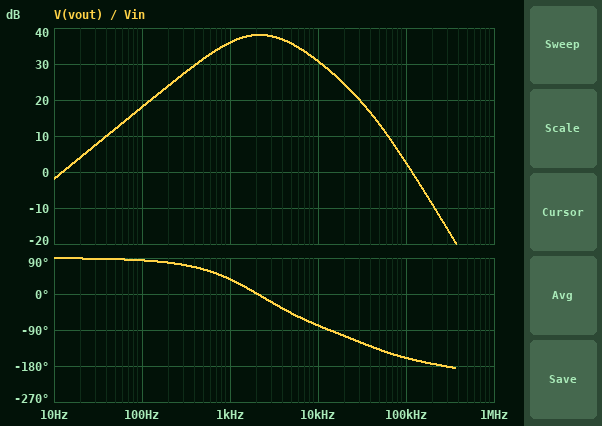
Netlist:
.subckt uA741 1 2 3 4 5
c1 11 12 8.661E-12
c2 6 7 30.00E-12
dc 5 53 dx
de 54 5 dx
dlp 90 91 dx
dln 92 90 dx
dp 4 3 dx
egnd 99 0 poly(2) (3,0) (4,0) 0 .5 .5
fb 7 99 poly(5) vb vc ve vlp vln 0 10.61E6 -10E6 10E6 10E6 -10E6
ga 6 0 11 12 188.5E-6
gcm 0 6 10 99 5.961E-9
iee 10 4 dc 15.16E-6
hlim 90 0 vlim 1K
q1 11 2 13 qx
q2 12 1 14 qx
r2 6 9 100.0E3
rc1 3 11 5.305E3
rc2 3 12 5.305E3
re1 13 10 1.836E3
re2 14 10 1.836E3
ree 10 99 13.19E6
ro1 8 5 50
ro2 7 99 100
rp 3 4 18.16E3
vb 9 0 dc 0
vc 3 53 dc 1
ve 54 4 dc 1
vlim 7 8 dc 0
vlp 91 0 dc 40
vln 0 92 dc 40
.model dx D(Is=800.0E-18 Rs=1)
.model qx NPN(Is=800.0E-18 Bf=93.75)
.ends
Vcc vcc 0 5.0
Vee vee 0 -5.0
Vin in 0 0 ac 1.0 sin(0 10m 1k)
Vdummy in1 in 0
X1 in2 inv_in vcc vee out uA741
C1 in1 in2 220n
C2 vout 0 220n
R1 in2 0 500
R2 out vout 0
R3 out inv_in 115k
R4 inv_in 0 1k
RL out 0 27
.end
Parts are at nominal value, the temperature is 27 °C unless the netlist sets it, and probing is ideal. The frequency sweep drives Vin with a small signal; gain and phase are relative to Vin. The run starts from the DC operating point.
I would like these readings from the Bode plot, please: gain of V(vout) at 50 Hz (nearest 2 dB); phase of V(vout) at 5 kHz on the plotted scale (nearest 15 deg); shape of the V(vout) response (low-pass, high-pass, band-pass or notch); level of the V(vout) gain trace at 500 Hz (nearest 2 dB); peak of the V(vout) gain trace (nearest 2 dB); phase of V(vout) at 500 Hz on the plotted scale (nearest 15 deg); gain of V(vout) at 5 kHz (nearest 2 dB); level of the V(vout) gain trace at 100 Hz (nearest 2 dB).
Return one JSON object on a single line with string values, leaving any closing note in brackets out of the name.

{"gain of V(vout) at 50 Hz": "12 dB", "phase of V(vout) at 5 kHz on the plotted scale": "-45 deg", "shape of the V(vout) response": "band-pass", "level of the V(vout) gain trace at 500 Hz": "32 dB", "peak of the V(vout) gain trace": "38 dB", "phase of V(vout) at 500 Hz on the plotted scale": "60 deg", "gain of V(vout) at 5 kHz": "36 dB", "level of the V(vout) gain trace at 100 Hz": "18 dB"}
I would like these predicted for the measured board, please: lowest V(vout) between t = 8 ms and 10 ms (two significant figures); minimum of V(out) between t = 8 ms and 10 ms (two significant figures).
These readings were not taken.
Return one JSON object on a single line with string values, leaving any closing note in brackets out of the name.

{"lowest V(vout) between t = 8 ms and 10 ms": "-620 mV", "minimum of V(out) between t = 8 ms and 10 ms": "-620 mV"}
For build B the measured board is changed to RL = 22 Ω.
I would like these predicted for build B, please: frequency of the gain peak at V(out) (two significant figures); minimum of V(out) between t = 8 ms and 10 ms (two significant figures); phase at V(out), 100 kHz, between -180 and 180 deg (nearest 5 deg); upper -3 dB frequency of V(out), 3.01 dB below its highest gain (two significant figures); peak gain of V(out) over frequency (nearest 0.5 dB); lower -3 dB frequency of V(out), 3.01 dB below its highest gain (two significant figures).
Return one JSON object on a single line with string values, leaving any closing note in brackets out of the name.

{"frequency of the gain peak at V(out)": "2.0 kHz", "minimum of V(out) between t = 8 ms and 10 ms": "-610 mV", "phase at V(out), 100 kHz, between -180 and 180 deg": "-155 deg", "upper -3 dB frequency of V(out), 3.01 dB below its highest gain": "5.0 kHz", "peak gain of V(out) over frequency": "37.5 dB", "lower -3 dB frequency of V(out), 3.01 dB below its highest gain": "800 Hz"}
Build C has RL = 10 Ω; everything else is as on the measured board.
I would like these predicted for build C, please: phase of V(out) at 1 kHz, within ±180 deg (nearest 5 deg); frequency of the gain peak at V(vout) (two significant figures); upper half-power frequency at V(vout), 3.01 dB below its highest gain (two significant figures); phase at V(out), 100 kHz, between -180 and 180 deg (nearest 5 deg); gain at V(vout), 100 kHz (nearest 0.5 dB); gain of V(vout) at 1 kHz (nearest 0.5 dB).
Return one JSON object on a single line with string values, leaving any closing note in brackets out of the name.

{"phase of V(out) at 1 kHz, within ±180 deg": "20 deg", "frequency of the gain peak at V(vout)": "1.5 kHz", "upper half-power frequency at V(vout), 3.01 dB below its highest gain": "3.5 kHz", "phase at V(out), 100 kHz, between -180 and 180 deg": "-140 deg", "gain at V(vout), 100 kHz": "1.0 dB", "gain of V(vout) at 1 kHz": "34.5 dB"}
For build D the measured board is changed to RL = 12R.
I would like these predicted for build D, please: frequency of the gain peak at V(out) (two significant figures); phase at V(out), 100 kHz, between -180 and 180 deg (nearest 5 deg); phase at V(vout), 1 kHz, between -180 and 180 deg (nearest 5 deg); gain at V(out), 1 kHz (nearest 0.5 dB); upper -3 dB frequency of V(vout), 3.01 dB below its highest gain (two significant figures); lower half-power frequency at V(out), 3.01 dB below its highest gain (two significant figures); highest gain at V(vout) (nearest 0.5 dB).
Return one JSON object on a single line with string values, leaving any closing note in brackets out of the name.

{"frequency of the gain peak at V(out)": "1.6 kHz", "phase at V(out), 100 kHz, between -180 and 180 deg": "-145 deg", "phase at V(vout), 1 kHz, between -180 and 180 deg": "25 deg", "gain at V(out), 1 kHz": "35.0 dB", "upper -3 dB frequency of V(vout), 3.01 dB below its highest gain": "3.8 kHz", "lower half-power frequency at V(out), 3.01 dB below its highest gain": "650 Hz", "highest gain at V(vout)": "36.0 dB"}
